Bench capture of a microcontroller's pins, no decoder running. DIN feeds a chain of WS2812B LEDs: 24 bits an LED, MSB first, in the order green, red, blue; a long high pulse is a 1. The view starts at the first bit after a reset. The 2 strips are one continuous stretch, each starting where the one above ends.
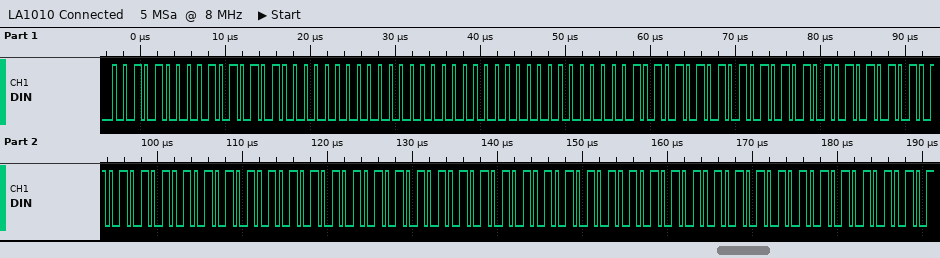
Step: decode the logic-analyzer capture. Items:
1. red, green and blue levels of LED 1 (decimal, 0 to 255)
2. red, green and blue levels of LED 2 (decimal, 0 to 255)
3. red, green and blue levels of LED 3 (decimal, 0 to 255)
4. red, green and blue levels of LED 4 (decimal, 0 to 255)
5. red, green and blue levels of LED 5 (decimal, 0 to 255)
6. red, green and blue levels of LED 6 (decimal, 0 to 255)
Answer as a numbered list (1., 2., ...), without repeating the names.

1. 85, 40, 0
2. 0, 0, 0
3. 85, 85, 85
4. 85, 85, 85
5. 85, 85, 85
6. 85, 85, 85
